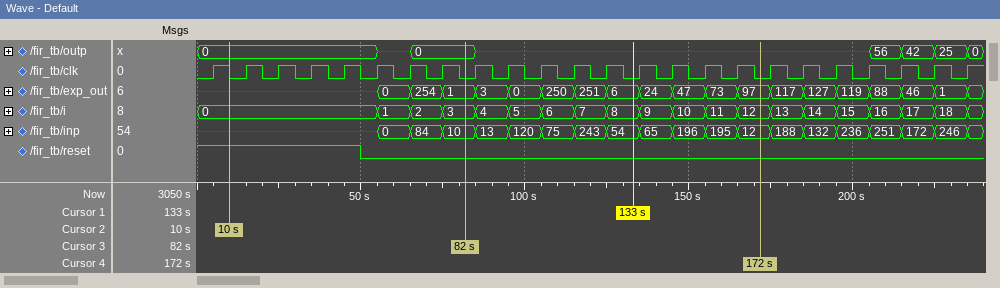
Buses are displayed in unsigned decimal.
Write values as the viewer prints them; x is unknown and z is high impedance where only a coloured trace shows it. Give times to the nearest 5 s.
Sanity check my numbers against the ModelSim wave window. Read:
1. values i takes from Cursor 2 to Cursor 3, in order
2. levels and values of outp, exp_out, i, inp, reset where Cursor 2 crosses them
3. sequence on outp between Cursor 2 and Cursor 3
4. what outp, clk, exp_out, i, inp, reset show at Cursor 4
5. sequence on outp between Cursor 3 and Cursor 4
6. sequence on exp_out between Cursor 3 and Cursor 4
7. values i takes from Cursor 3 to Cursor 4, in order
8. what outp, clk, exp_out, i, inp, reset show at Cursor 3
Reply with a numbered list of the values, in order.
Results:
1. 0, 1, 2, 3
2. outp=0, exp_out=x, i=0, inp=x, reset=1
3. 0, x, 0
4. outp=x, clk=0, exp_out=97, i=12, inp=12, reset=0
5. 0, x
6. 1, 3, 0, 250, 251, 6, 24, 47, 73, 97
7. 3, 4, 5, 6, 7, 8, 9, 10, 11, 12
8. outp=0, clk=0, exp_out=1, i=3, inp=10, reset=0
